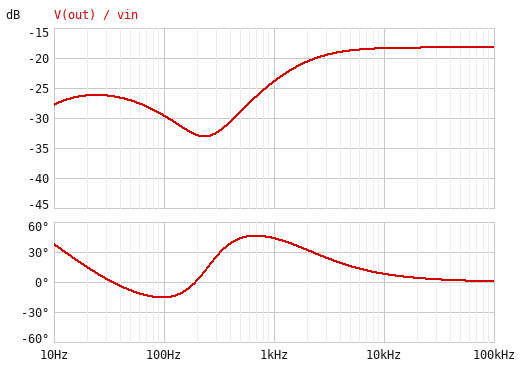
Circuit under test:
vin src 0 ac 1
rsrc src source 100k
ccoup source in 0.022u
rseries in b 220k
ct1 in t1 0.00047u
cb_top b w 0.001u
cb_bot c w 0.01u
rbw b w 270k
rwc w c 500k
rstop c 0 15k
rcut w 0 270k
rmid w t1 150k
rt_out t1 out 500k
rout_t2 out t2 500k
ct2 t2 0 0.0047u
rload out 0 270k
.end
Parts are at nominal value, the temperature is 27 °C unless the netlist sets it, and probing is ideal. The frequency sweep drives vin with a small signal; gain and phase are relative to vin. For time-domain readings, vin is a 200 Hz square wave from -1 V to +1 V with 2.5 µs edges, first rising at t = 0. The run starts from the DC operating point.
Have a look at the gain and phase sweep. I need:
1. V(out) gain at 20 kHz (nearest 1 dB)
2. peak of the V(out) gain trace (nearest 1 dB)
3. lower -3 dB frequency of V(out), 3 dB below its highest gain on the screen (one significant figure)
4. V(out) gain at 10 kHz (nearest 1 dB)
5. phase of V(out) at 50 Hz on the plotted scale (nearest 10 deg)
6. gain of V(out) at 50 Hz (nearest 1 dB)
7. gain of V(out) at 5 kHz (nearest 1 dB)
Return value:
-18 dB
-18 dB
2 kHz
-18 dB
-10 deg
-27 dB
-19 dB
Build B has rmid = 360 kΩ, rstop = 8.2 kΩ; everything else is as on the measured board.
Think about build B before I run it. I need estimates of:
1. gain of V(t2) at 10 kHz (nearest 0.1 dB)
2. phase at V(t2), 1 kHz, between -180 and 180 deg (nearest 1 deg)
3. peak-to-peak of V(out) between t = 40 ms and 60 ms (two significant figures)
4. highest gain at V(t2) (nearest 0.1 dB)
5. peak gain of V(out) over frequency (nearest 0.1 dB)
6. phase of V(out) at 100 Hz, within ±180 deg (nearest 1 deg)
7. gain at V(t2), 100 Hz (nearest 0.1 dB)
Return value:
-60.4 dB
-47 deg
510 mV
-28.2 dB
-17.0 dB
-1 deg
-36.6 dB
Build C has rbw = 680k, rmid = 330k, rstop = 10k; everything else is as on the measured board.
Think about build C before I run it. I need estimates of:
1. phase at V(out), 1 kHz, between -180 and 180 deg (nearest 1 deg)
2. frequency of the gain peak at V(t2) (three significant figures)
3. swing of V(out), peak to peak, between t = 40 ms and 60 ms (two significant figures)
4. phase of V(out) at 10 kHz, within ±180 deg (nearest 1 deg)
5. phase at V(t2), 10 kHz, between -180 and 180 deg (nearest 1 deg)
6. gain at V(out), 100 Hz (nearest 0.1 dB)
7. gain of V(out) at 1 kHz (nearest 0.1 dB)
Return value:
38 deg
16.4 Hz
520 mV
5 deg
-84 deg
-32.8 dB
-20.3 dB
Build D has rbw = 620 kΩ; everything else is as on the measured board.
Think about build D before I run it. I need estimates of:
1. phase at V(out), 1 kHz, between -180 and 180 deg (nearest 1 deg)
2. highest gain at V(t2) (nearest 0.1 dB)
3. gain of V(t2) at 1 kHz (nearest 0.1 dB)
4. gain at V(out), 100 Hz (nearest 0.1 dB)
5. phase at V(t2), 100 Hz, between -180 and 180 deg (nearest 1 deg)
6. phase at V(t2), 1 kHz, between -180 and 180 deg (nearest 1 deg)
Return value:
42 deg
-29.4 dB
-47.2 dB
-32.0 dB
-57 deg
-44 deg
